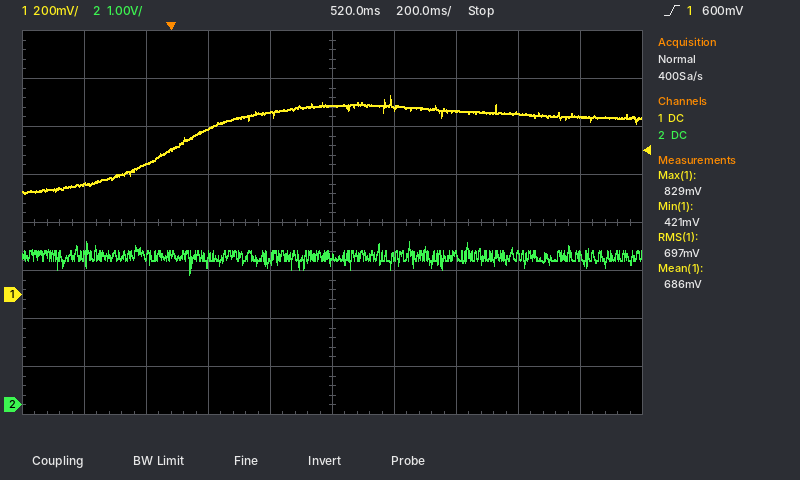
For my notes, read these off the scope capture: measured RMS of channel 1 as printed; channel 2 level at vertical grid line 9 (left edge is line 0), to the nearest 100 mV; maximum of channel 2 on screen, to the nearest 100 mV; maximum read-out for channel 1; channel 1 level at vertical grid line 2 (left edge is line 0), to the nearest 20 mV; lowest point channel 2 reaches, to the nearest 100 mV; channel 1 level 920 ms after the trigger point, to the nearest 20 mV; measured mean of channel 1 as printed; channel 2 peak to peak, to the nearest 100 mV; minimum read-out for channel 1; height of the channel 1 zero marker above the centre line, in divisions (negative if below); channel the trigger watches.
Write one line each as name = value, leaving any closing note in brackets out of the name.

measured RMS of channel 1 as printed = 697 mV
channel 2 level at vertical grid line 9 (left edge is line 0), to the nearest 100 mV = 3.1 V
maximum of channel 2 on screen, to the nearest 100 mV = 3.4 V
maximum read-out for channel 1 = 829 mV
channel 1 level at vertical grid line 2 (left edge is line 0), to the nearest 20 mV = 540 mV
lowest point channel 2 reaches, to the nearest 100 mV = 2.7 V
channel 1 level 920 ms after the trigger point, to the nearest 20 mV = 760 mV
measured mean of channel 1 as printed = 686 mV
channel 2 peak to peak, to the nearest 100 mV = 700 mV
minimum read-out for channel 1 = 421 mV
height of the channel 1 zero marker above the centre line, in divisions = -1.5 div
channel the trigger watches = channel 1
